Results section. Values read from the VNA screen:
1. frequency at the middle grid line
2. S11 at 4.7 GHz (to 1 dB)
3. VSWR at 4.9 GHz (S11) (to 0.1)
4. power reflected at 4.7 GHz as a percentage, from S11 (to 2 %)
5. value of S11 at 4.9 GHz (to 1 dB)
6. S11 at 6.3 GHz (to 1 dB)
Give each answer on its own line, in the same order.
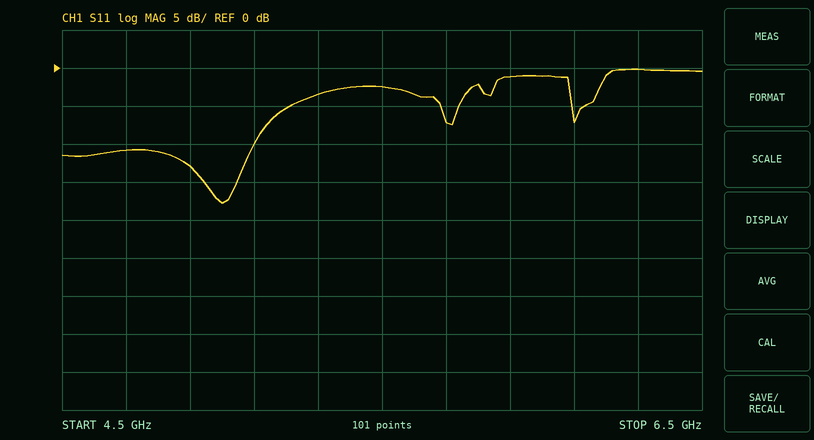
5.5 GHz
-11 dB
1.6
8 %
-13 dB
0 dB
